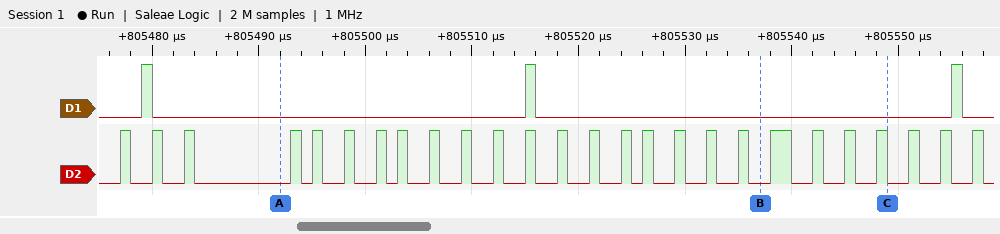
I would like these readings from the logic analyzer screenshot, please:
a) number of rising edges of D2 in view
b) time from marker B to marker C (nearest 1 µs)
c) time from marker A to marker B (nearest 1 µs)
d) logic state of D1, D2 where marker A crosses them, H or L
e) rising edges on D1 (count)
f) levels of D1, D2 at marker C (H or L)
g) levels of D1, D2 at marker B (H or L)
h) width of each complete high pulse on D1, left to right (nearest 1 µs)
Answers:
26
12 µs
45 µs
D1=L, D2=L
3
D1=L, D2=L
D1=L, D2=L
1 µs, 1 µs, 1 µs
